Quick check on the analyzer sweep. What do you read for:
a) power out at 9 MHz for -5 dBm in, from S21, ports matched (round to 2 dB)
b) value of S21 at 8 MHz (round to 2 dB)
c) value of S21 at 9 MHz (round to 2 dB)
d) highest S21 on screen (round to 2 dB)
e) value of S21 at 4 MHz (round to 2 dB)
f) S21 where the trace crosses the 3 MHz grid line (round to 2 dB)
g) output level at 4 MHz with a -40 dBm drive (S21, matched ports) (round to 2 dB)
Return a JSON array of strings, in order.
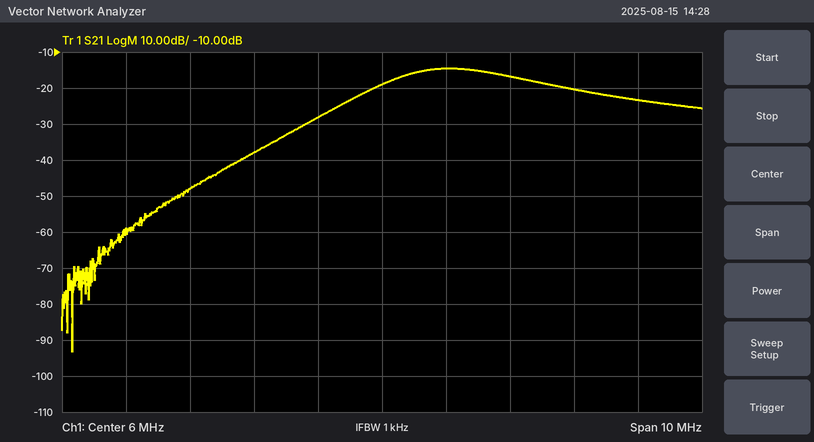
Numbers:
["-26 dBm", "-16 dB", "-20 dB", "-14 dB", "-38 dB", "-48 dB", "-78 dBm"]
